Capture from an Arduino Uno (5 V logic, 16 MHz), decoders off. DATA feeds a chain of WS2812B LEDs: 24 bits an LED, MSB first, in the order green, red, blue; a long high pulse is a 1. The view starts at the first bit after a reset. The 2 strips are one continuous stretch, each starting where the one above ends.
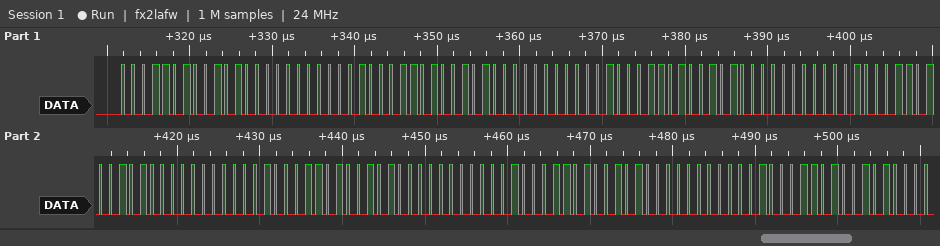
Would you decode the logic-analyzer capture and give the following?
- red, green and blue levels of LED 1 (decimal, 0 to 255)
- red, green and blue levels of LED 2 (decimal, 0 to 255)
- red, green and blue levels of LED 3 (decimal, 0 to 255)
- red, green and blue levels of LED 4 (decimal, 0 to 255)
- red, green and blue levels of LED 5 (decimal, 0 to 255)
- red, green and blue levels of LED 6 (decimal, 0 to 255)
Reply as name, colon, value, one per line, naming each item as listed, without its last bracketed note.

red, green and blue levels of LED 1: 80, 26, 1
red, green and blue levels of LED 2: 80, 26, 1
red, green and blue levels of LED 3: 80, 26, 1
red, green and blue levels of LED 4: 80, 26, 1
red, green and blue levels of LED 5: 80, 26, 1
red, green and blue levels of LED 6: 80, 26, 1
